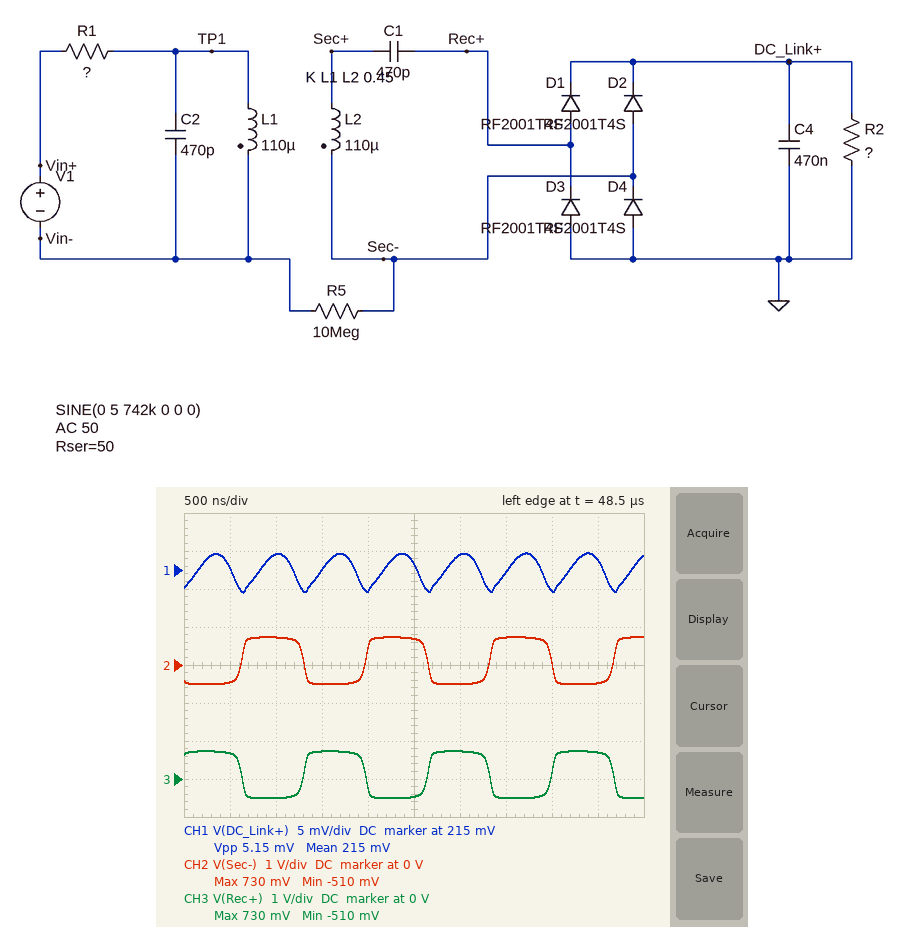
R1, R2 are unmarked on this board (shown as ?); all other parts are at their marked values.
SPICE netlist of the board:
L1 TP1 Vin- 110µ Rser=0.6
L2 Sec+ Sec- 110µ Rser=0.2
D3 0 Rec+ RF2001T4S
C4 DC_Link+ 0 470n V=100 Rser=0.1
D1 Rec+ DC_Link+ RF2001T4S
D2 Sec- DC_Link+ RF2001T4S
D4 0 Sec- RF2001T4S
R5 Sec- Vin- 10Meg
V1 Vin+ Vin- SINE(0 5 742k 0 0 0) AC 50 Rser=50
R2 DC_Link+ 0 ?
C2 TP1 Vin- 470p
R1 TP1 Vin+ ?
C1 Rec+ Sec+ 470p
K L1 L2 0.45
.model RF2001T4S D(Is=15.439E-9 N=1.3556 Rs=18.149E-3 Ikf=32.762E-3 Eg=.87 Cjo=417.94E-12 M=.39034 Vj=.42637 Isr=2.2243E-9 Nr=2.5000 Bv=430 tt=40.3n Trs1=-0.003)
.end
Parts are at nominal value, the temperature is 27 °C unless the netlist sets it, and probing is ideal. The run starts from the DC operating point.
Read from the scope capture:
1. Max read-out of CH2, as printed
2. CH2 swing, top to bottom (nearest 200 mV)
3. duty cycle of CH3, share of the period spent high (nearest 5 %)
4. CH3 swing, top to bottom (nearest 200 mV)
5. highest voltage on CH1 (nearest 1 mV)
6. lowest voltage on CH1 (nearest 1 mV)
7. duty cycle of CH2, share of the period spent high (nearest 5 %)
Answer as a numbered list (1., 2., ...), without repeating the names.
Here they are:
1. 730 mV
2. 1.2 V
3. 50 %
4. 1.2 V
5. 217 mV
6. 212 mV
7. 50 %
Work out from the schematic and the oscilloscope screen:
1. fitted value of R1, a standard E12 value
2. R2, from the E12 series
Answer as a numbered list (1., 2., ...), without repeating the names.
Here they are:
1. 27 Ω
2. 22 Ω
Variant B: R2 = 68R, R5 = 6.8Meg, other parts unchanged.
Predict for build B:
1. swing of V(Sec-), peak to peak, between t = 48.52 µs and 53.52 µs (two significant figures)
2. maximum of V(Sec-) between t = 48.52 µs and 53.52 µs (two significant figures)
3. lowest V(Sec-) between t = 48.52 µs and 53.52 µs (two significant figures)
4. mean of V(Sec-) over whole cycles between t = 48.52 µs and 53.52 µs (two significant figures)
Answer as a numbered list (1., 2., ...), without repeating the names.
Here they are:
1. 1.4 V
2. 910 mV
3. -500 mV
4. 210 mV
